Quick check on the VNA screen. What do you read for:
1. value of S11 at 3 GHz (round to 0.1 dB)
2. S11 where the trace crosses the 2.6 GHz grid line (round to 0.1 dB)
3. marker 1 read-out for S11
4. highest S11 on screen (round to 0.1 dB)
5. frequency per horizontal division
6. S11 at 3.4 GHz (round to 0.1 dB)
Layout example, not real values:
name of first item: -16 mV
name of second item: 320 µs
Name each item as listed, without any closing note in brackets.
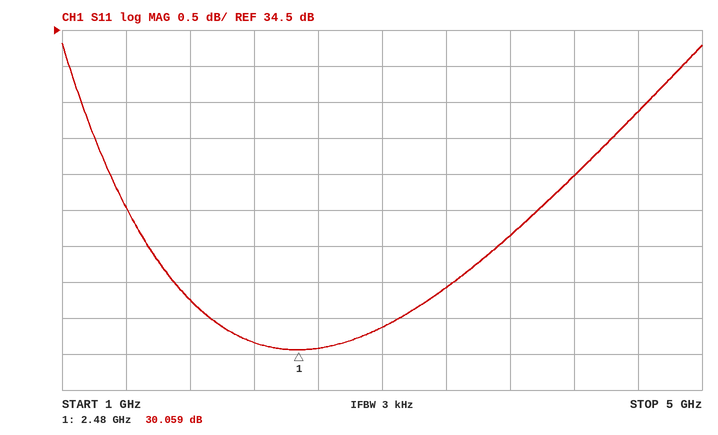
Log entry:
value of S11 at 3 GHz: 30.4 dB
S11 where the trace crosses the 2.6 GHz grid line: 30.1 dB
marker 1 read-out for S11: 30.059 dB
highest S11 on screen: 34.3 dB
frequency per horizontal division: 400 MHz
S11 at 3.4 GHz: 30.9 dB
